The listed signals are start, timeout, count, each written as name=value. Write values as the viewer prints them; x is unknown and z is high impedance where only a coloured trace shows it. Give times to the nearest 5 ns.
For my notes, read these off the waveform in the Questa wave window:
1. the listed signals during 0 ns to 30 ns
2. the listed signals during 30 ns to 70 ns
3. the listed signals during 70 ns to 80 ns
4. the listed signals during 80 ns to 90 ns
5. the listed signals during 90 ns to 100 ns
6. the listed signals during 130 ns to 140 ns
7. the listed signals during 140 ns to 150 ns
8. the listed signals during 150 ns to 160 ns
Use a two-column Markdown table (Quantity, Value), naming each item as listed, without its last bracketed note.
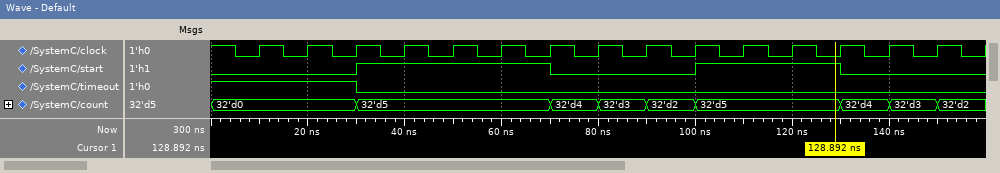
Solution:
| Quantity | Value |
|---|---|
| the listed signals during 0 ns to 30 ns | start=0, timeout=1, count=32'd0 |
| the listed signals during 30 ns to 70 ns | start=1, timeout=0, count=32'd5 |
| the listed signals during 70 ns to 80 ns | start=0, timeout=0, count=32'd4 |
| the listed signals during 80 ns to 90 ns | start=0, timeout=0, count=32'd3 |
| the listed signals during 90 ns to 100 ns | start=0, timeout=0, count=32'd2 |
| the listed signals during 130 ns to 140 ns | start=0, timeout=0, count=32'd4 |
| the listed signals during 140 ns to 150 ns | start=0, timeout=0, count=32'd3 |
| the listed signals during 150 ns to 160 ns | start=0, timeout=0, count=32'd2 |
